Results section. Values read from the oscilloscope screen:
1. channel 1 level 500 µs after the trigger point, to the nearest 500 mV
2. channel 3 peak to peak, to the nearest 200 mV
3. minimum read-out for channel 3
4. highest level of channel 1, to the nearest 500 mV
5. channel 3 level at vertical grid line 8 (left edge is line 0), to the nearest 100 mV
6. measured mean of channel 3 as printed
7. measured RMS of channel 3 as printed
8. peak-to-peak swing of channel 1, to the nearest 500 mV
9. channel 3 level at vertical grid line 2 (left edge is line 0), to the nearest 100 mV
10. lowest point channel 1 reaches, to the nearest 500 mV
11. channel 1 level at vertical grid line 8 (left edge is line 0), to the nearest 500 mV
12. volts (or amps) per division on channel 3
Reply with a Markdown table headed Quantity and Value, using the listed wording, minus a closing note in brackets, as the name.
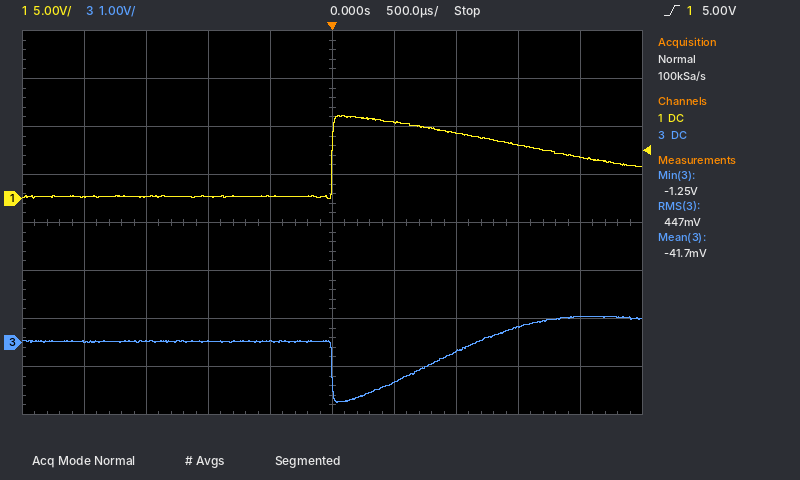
| Quantity | Value |
|---|---|
| channel 1 level 500 µs after the trigger point, to the nearest 500 mV | 8.0 V |
| channel 3 peak to peak, to the nearest 200 mV | 1.8 V |
| minimum read-out for channel 3 | -1.25 V |
| highest level of channel 1, to the nearest 500 mV | 8.5 V |
| channel 3 level at vertical grid line 8 (left edge is line 0), to the nearest 100 mV | 300 mV |
| measured mean of channel 3 as printed | -41.7 mV |
| measured RMS of channel 3 as printed | 447 mV |
| peak-to-peak swing of channel 1, to the nearest 500 mV | 8.5 V |
| channel 3 level at vertical grid line 2 (left edge is line 0), to the nearest 100 mV | 0.0 V |
| lowest point channel 1 reaches, to the nearest 500 mV | 0.0 V |
| channel 1 level at vertical grid line 8 (left edge is line 0), to the nearest 500 mV | 5.5 V |
| volts (or amps) per division on channel 3 | 1 V |
